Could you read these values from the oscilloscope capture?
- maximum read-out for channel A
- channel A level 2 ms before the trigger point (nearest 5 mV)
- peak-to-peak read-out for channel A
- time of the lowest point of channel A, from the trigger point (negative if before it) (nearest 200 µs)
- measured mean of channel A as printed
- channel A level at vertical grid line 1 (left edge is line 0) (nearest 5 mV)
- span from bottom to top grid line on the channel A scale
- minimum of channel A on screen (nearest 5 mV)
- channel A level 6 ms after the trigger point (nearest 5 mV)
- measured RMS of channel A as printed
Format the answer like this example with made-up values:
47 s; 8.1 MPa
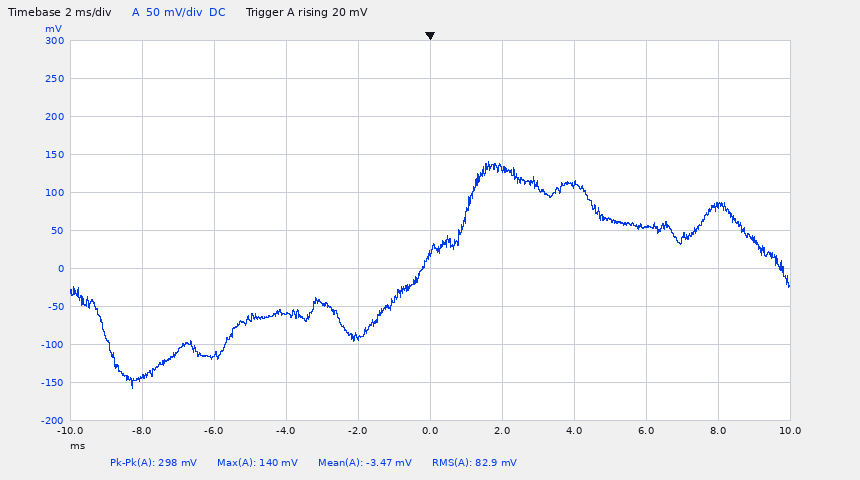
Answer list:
140 mV; -90 mV; 298 mV; -8.2 ms; -3.47 mV; -145 mV; 500 mV; -160 mV; 55 mV; 82.9 mV
